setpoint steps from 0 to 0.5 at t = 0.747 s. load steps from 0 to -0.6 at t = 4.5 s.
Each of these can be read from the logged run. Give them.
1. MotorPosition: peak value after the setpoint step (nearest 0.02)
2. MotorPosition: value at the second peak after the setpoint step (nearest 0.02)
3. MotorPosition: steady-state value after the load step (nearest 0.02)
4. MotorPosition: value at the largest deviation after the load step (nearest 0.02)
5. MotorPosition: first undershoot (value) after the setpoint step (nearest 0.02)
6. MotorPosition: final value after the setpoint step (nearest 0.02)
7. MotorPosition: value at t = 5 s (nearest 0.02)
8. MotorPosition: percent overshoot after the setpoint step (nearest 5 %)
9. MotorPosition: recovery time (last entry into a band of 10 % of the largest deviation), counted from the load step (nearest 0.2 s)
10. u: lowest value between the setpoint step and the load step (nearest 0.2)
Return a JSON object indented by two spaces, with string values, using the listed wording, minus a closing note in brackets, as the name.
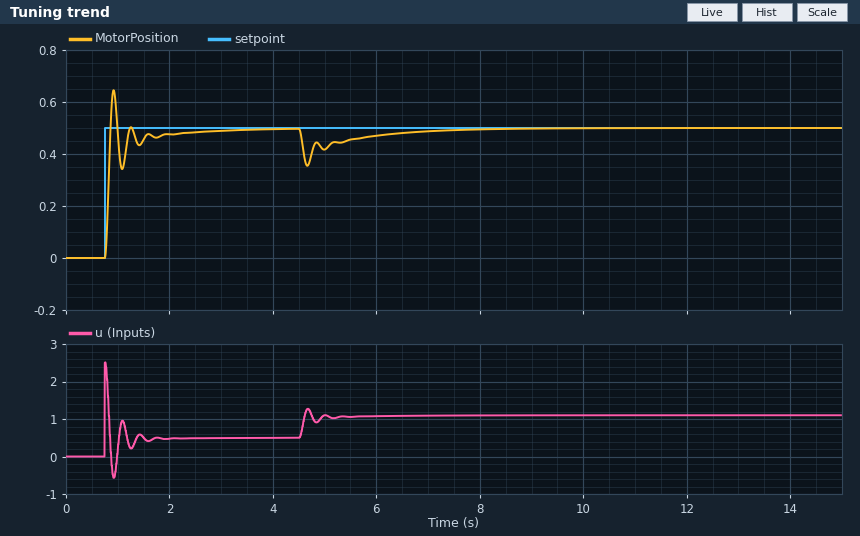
{
  "MotorPosition: peak value after the setpoint step": "0.64",
  "MotorPosition: value at the second peak after the setpoint step": "0.50",
  "MotorPosition: steady-state value after the load step": "0.50",
  "MotorPosition: value at the largest deviation after the load step": "0.36",
  "MotorPosition: first undershoot (value) after the setpoint step": "0.34",
  "MotorPosition: final value after the setpoint step": "0.50",
  "MotorPosition: value at t = 5 s": "0.42",
  "MotorPosition: percent overshoot after the setpoint step": "30 %",
  "MotorPosition: recovery time (last entry into a band of 10 % of the largest deviation), counted from the load step": "2.4 s",
  "u: lowest value between the setpoint step and the load step": "-0.6"
}
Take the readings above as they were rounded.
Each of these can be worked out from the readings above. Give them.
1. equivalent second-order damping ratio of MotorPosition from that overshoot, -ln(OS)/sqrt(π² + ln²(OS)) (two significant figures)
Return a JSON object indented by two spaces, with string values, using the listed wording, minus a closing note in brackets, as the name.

{
  "equivalent second-order damping ratio of MotorPosition from that overshoot, -ln(OS)/sqrt(π² + ln²(OS))": "0.36"
}
